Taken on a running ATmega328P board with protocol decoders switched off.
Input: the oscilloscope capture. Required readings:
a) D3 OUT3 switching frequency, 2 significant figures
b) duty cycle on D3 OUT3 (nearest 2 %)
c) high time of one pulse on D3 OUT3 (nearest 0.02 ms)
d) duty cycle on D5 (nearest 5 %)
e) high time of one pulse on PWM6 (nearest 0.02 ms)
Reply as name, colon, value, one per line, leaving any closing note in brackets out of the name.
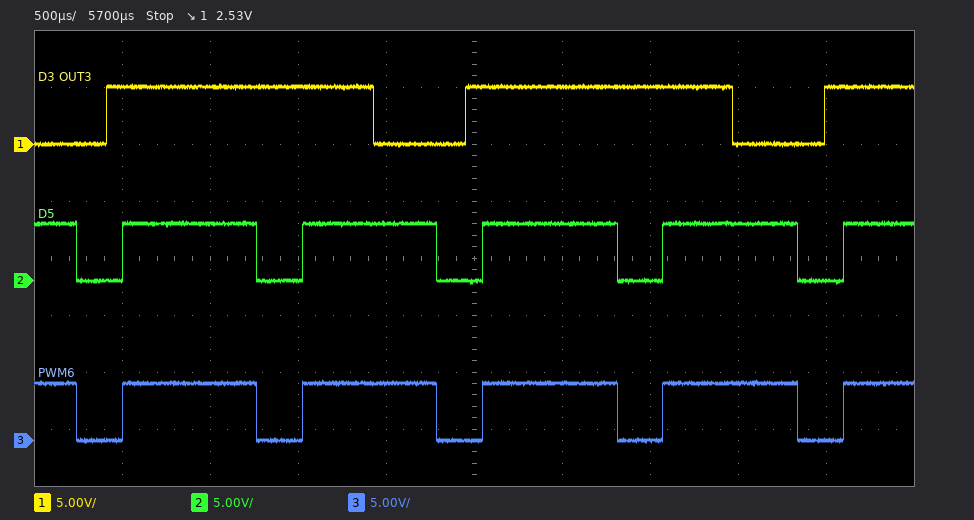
D3 OUT3 switching frequency, 2 significant figures: 490 Hz
duty cycle on D3 OUT3: 74 %
high time of one pulse on D3 OUT3: 1.52 ms
duty cycle on D5: 75 %
high time of one pulse on PWM6: 0.76 ms
